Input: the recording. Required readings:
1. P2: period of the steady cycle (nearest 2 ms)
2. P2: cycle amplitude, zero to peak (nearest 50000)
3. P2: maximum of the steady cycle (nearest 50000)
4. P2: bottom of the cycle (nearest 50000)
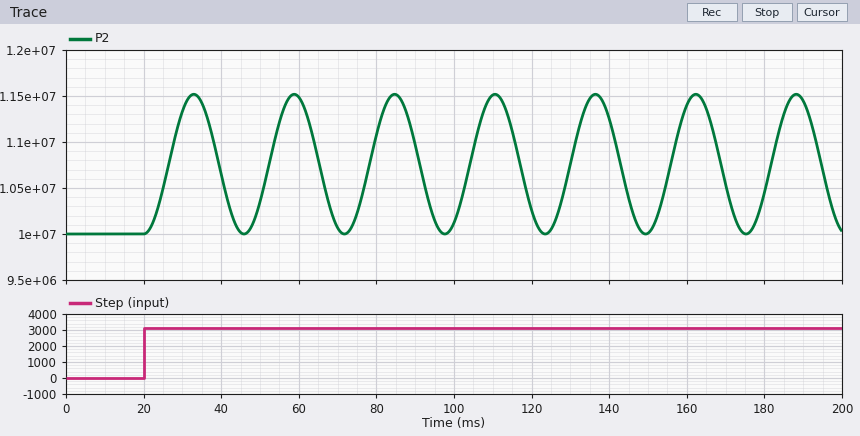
26 ms
750000
11500000
10000000
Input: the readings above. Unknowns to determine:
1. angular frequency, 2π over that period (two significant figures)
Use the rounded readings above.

0.24 rad/ms
